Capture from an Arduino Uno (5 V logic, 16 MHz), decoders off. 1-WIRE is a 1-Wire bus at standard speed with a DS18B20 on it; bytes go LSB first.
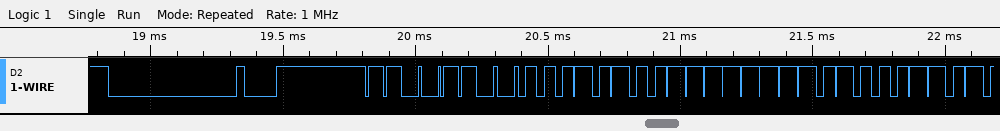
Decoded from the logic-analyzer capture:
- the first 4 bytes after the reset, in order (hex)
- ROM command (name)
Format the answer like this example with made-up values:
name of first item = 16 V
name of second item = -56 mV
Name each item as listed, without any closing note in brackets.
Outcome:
the first 4 bytes after the reset, in order = 33 28 FF 62
ROM command = Read ROM
